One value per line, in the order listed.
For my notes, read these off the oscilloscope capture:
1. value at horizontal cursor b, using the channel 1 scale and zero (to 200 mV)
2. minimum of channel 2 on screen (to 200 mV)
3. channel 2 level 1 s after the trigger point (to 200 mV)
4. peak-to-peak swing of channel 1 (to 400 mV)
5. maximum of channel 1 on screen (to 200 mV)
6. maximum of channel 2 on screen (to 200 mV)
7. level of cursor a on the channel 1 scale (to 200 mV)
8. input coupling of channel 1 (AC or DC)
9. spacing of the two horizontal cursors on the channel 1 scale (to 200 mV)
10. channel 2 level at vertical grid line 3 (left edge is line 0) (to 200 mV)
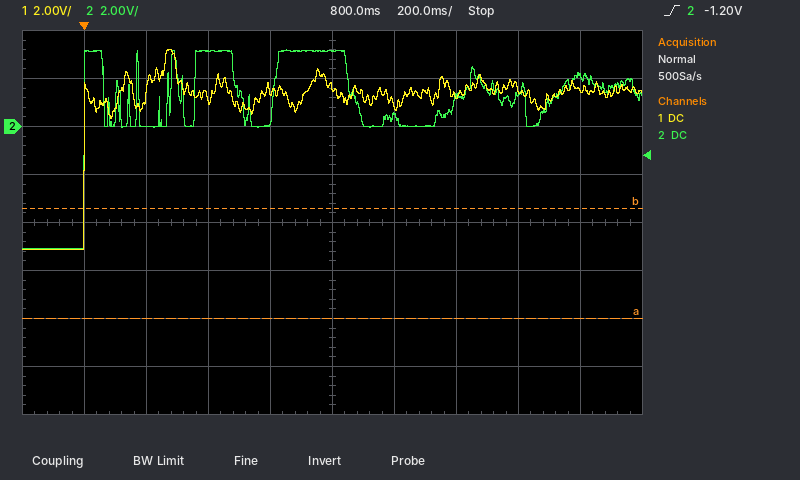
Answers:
-3.4 V
-5.0 V
400 mV
8.4 V
3.2 V
3.2 V
-8.0 V
DC
4.6 V
3.2 V
